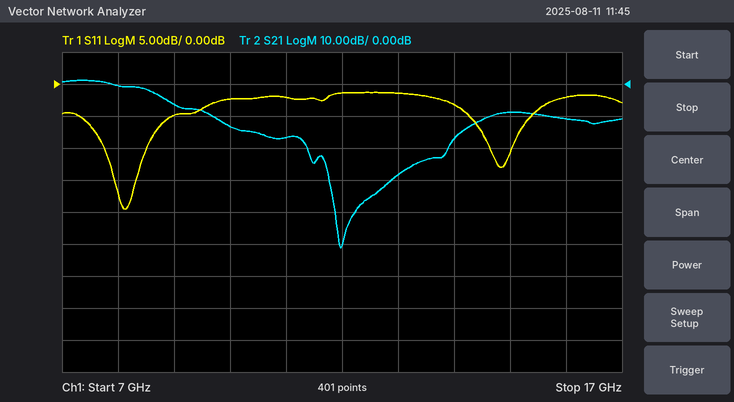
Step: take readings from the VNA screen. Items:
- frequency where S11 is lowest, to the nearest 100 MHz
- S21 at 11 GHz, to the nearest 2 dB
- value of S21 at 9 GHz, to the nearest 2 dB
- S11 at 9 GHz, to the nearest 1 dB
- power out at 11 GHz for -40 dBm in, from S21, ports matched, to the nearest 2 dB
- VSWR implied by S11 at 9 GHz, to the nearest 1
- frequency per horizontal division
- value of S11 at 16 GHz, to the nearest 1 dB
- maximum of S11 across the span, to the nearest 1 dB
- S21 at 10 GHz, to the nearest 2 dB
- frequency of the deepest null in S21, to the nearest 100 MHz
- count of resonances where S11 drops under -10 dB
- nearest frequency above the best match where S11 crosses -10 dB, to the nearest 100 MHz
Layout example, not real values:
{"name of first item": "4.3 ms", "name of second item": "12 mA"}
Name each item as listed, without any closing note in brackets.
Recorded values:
{"frequency where S11 is lowest, to the nearest 100 MHz": "8.1 GHz", "S21 at 11 GHz, to the nearest 2 dB": "-16 dB", "value of S21 at 9 GHz, to the nearest 2 dB": "-6 dB", "S11 at 9 GHz, to the nearest 1 dB": "-5 dB", "power out at 11 GHz for -40 dBm in, from S21, ports matched, to the nearest 2 dB": "-56 dBm", "VSWR implied by S11 at 9 GHz, to the nearest 1": "4", "frequency per horizontal division": "1 GHz", "value of S11 at 16 GHz, to the nearest 1 dB": "-2 dB", "maximum of S11 across the span, to the nearest 1 dB": "-1 dB", "S21 at 10 GHz, to the nearest 2 dB": "-14 dB", "frequency of the deepest null in S21, to the nearest 100 MHz": "12.0 GHz", "count of resonances where S11 drops under -10 dB": "2", "nearest frequency above the best match where S11 crosses -10 dB, to the nearest 100 MHz": "8.5 GHz"}
